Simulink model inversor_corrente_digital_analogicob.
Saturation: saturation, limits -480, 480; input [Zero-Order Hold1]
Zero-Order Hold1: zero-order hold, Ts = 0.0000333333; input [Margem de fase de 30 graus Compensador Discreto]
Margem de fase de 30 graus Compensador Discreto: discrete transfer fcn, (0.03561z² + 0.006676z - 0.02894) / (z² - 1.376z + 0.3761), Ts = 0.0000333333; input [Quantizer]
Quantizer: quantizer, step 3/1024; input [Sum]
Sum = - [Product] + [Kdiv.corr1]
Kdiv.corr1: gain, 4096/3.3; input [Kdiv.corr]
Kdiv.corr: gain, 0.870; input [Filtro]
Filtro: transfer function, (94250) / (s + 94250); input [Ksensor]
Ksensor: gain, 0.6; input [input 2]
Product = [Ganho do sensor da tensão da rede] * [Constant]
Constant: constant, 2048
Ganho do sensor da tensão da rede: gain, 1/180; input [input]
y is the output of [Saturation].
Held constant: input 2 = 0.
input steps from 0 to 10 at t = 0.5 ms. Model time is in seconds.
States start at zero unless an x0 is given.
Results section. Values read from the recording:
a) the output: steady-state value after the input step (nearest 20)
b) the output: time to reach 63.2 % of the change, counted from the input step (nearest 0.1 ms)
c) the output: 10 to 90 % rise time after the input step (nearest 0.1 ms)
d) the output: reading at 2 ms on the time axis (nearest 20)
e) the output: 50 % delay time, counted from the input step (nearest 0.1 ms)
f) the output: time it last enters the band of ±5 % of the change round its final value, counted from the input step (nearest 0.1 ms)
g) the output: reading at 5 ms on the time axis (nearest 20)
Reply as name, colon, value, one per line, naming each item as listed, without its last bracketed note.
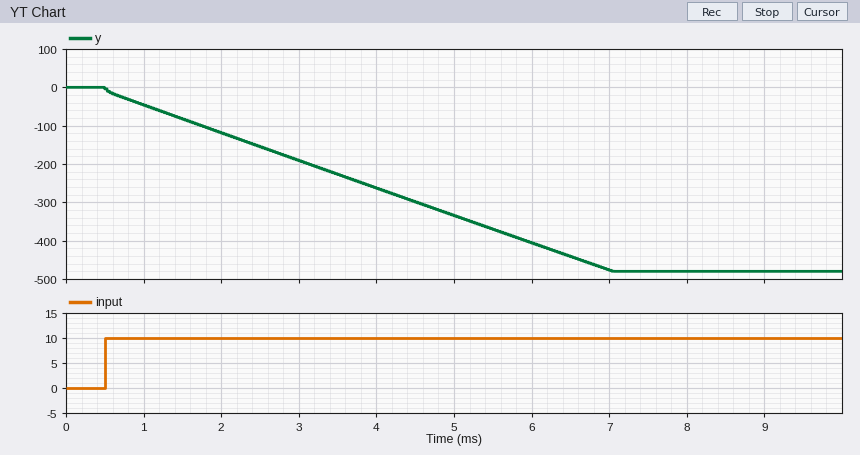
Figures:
the output: steady-state value after the input step: -480
the output: time to reach 63.2 % of the change, counted from the input step: 4.1 ms
the output: 10 to 90 % rise time after the input step: 5.3 ms
the output: reading at 2 ms on the time axis: -120
the output: 50 % delay time, counted from the input step: 3.2 ms
the output: time it last enters the band of ±5 % of the change round its final value, counted from the input step: 6.2 ms
the output: reading at 5 ms on the time axis: -340
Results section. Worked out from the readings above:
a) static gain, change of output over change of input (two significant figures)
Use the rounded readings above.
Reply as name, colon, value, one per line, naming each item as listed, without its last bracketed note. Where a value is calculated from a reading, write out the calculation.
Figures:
static gain, change of output over change of input: (-480 - 0) / (10 - 0) = -48
